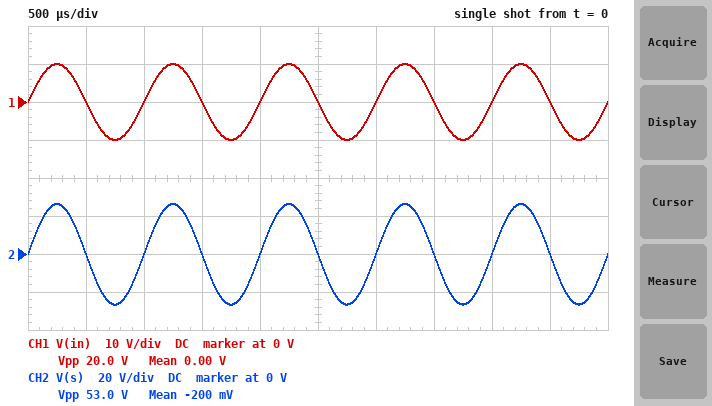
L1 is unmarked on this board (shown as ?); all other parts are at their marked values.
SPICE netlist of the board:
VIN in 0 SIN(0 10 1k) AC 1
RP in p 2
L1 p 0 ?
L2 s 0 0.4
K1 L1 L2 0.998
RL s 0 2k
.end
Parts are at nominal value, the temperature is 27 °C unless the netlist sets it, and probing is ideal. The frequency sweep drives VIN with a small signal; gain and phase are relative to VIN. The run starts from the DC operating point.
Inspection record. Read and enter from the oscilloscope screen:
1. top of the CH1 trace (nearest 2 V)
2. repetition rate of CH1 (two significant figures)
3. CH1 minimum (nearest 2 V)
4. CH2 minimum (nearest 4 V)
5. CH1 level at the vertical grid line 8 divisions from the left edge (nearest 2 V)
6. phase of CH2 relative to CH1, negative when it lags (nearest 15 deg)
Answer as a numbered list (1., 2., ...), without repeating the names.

1. 10 V
2. 1.0 kHz
3. -10 V
4. -28 V
5. 0 V
6. 0 deg
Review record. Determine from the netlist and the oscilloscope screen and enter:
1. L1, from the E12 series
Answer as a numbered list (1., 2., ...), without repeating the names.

1. 56 mH
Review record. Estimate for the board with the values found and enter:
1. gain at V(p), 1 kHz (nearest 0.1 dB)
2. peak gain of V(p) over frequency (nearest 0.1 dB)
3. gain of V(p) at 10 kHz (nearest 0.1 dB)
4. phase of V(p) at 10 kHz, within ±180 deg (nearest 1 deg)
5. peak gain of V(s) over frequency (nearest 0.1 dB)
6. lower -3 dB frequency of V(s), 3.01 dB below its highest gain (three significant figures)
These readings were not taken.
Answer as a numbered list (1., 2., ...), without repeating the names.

1. -0.1 dB
2. 0 dB
3. -0.1 dB
4. 0 deg
5. 8.5 dB
6. 5.64 Hz
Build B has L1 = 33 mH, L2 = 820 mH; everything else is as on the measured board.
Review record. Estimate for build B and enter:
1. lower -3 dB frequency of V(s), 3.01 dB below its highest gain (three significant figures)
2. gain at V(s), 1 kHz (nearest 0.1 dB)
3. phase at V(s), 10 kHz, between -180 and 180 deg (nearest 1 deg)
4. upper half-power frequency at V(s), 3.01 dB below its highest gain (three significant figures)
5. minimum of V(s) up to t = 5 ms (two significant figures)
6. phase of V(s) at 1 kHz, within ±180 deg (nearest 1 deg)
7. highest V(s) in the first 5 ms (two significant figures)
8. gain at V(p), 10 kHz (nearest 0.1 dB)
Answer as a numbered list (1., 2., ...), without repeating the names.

1. 9.41 Hz
2. 13.7 dB
3. -6 deg
4. 99.6 kHz
5. -49 V
6. 0 deg
7. 48 V
8. -0.2 dB
